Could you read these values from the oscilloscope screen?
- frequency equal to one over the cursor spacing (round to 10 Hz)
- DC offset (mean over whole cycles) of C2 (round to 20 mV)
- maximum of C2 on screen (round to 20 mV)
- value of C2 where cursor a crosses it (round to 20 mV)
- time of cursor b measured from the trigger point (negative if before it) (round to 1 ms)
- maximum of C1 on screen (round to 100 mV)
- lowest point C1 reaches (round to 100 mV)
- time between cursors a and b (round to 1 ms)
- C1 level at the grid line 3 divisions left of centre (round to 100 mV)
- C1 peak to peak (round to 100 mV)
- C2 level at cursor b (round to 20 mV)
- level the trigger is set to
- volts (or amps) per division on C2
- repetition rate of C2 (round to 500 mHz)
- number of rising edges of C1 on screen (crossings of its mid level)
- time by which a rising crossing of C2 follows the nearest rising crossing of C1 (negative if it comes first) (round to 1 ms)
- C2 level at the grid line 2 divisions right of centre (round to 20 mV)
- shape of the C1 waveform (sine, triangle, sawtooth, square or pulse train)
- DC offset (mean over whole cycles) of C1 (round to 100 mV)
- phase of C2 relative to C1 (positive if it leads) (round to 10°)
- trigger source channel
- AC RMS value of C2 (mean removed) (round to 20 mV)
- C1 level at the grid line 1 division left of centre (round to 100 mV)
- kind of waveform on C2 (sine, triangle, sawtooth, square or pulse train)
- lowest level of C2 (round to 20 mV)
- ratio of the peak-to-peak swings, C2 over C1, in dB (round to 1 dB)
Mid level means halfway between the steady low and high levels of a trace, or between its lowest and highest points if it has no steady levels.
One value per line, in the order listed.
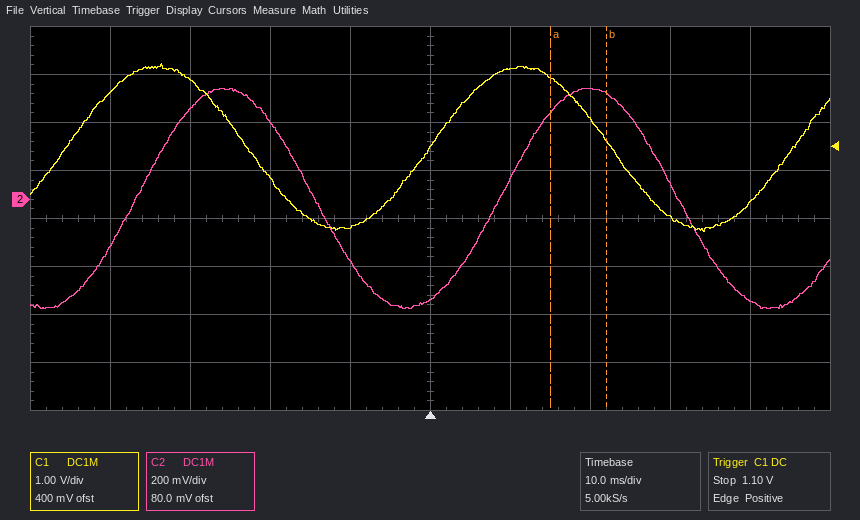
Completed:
140 Hz
0 mV
460 mV
360 mV
+22 ms
2.8 V
-700 mV
7 ms
2.5 V
3.5 V
440 mV
1.10 V
200 mV
22.0 Hz
3
+9 ms
460 mV
sine
1.1 V
-70°
C1
320 mV
-600 mV
sine
-460 mV
-12 dB
